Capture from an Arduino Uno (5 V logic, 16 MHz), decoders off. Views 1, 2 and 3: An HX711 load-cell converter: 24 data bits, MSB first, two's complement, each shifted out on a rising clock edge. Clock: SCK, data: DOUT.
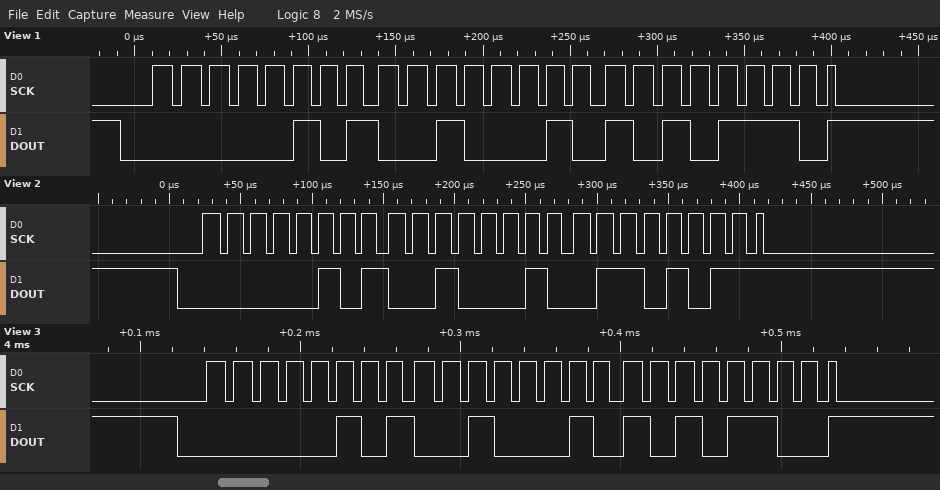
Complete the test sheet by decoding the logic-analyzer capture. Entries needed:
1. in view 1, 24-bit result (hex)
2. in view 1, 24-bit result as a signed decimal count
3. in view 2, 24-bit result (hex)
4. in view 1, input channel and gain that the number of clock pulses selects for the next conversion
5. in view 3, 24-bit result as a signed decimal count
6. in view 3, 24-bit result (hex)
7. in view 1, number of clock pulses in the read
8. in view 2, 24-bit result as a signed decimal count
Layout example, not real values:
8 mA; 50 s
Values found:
0x0522AE; 336558; 0x05226B; channel A, gain 128; 336556; 0x0522AC; 25; 336491
